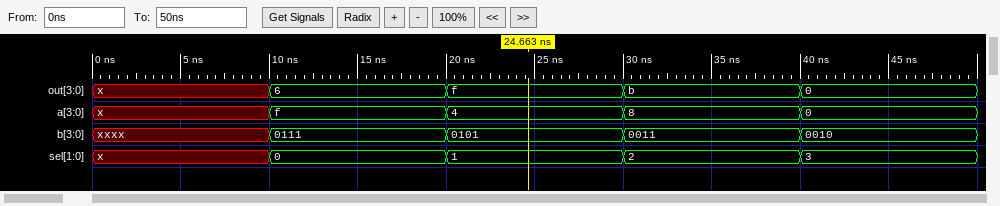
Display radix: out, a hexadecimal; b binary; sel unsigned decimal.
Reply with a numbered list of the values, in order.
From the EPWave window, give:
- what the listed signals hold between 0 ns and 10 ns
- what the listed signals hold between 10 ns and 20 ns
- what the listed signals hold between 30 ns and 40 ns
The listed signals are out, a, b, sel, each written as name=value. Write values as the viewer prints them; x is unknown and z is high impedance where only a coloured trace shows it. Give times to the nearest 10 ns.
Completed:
1. out=x, a=x, b=xxxx, sel=x
2. out=6, a=f, b=0111, sel=0
3. out=b, a=8, b=0011, sel=2
